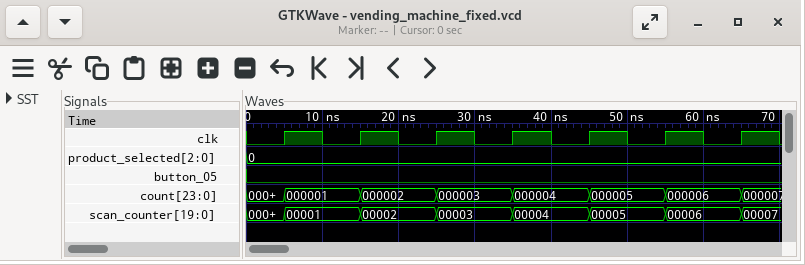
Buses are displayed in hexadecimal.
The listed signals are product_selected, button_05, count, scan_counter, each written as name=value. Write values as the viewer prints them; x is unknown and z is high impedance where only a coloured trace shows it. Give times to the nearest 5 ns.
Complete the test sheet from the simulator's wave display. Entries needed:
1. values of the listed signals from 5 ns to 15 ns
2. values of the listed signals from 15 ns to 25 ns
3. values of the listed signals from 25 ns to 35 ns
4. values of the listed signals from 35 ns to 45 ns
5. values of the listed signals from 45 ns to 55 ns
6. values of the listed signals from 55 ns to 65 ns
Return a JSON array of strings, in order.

["product_selected=0, button_05=0, count=000001, scan_counter=00001", "product_selected=0, button_05=0, count=000002, scan_counter=00002", "product_selected=0, button_05=0, count=000003, scan_counter=00003", "product_selected=0, button_05=0, count=000004, scan_counter=00004", "product_selected=0, button_05=0, count=000005, scan_counter=00005", "product_selected=0, button_05=0, count=000006, scan_counter=00006"]
